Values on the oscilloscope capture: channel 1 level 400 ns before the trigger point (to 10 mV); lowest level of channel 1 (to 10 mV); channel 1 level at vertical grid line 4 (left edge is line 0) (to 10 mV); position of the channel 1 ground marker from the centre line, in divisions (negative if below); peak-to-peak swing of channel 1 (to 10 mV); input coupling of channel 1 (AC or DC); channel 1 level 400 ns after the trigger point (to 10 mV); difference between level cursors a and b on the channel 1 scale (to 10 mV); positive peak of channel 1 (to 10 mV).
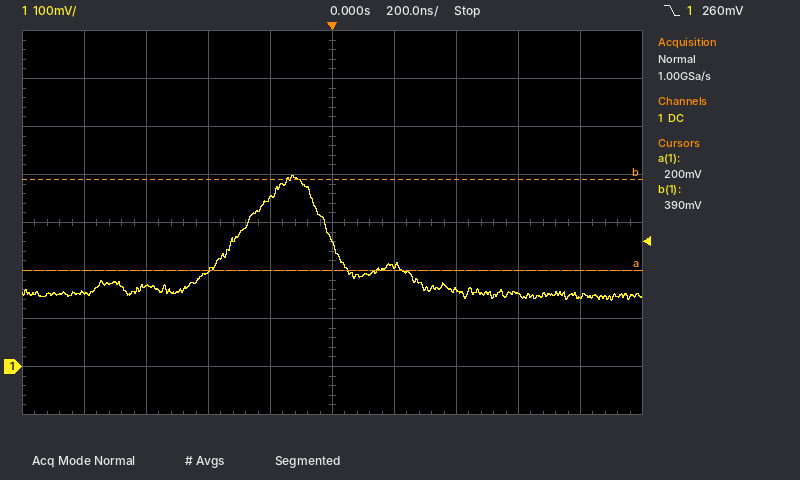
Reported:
200 mV
140 mV
350 mV
-3.0 div
260 mV
DC
160 mV
190 mV
400 mV
